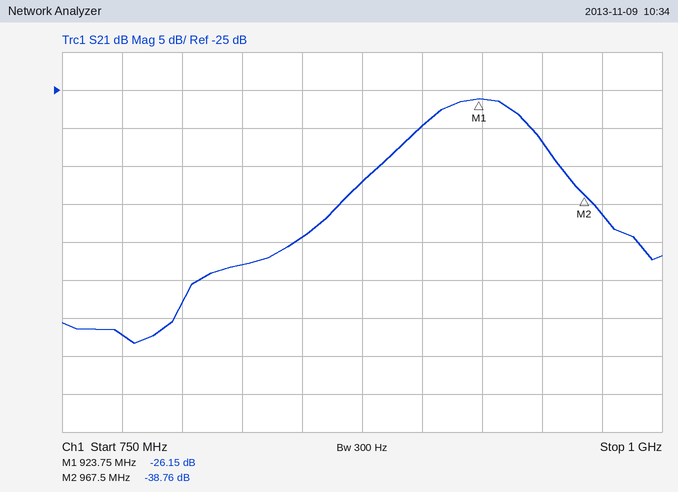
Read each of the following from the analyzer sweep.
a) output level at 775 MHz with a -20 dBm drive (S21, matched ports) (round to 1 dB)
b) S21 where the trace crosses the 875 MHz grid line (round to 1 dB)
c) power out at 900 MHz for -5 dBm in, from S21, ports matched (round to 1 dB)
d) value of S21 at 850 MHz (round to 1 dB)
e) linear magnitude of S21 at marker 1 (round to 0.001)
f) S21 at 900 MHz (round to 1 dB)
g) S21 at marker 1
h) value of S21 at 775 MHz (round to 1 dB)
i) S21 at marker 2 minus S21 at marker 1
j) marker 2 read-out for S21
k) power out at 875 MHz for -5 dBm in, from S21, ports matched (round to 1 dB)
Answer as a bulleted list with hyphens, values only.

- -77 dBm
- -37 dB
- -35 dBm
- -44 dB
- 0.049
- -30 dB
- -26.15 dB
- -57 dB
- -12.61 dB
- -38.76 dB
- -42 dBm
